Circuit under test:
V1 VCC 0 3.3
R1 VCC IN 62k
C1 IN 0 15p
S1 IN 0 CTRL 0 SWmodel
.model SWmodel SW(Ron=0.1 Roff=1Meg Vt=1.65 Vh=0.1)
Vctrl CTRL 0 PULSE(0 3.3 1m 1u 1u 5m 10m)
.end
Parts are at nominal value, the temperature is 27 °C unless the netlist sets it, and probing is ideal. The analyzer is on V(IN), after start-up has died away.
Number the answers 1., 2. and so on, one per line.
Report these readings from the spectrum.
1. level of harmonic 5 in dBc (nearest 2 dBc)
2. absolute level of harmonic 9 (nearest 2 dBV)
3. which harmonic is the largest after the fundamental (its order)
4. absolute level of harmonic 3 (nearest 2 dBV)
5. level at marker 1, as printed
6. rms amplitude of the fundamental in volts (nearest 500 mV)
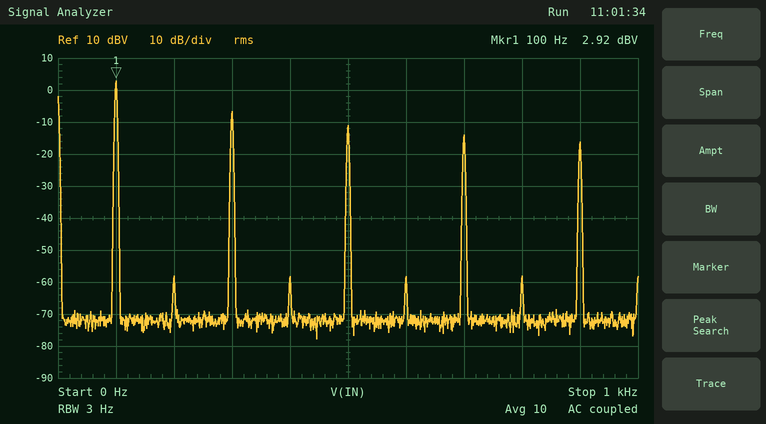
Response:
1. -14 dBc
2. -16 dBV
3. 3
4. -6 dBV
5. 2.92 dBV
6. 1.5 V
